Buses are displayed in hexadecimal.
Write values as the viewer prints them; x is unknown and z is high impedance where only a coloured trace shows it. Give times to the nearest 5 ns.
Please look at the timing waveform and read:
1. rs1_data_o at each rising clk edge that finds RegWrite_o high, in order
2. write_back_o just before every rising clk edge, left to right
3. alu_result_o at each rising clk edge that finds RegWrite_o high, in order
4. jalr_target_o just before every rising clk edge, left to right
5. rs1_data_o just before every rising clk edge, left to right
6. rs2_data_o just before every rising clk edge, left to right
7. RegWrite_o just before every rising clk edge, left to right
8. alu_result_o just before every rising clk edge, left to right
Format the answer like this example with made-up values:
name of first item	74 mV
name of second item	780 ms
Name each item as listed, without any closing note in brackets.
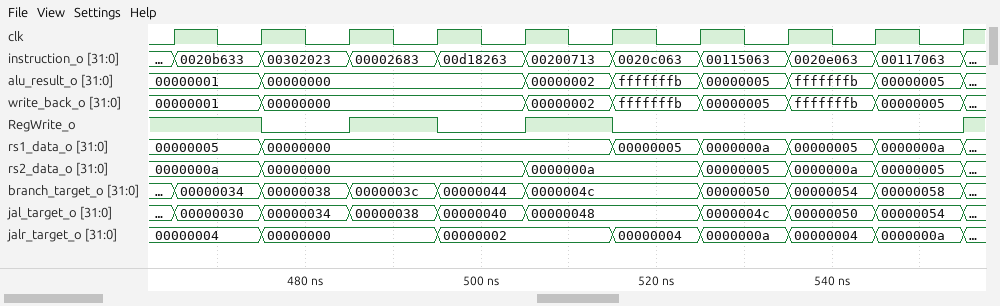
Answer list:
rs1_data_o at each rising clk edge that finds RegWrite_o high, in order	00000005, 00000005, 00000000, 00000000
write_back_o just before every rising clk edge, left to right	00000001, 00000001, 00000000, 00000000, 00000000, 00000002, fffffffb, 00000005, fffffffb, 00000005
alu_result_o at each rising clk edge that finds RegWrite_o high, in order	00000001, 00000001, 00000000, 00000002
jalr_target_o just before every rising clk edge, left to right	00000004, 00000004, 00000000, 00000000, 00000002, 00000002, 00000004, 0000000a, 00000004, 0000000a
rs1_data_o just before every rising clk edge, left to right	00000005, 00000005, 00000000, 00000000, 00000000, 00000000, 00000005, 0000000a, 00000005, 0000000a
rs2_data_o just before every rising clk edge, left to right	0000000a, 0000000a, 00000000, 00000000, 00000000, 0000000a, 0000000a, 00000005, 0000000a, 00000005
RegWrite_o just before every rising clk edge, left to right	1 1 0 1 0 1 0 0 0 0
alu_result_o just before every rising clk edge, left to right	00000001, 00000001, 00000000, 00000000, 00000000, 00000002, fffffffb, 00000005, fffffffb, 00000005
